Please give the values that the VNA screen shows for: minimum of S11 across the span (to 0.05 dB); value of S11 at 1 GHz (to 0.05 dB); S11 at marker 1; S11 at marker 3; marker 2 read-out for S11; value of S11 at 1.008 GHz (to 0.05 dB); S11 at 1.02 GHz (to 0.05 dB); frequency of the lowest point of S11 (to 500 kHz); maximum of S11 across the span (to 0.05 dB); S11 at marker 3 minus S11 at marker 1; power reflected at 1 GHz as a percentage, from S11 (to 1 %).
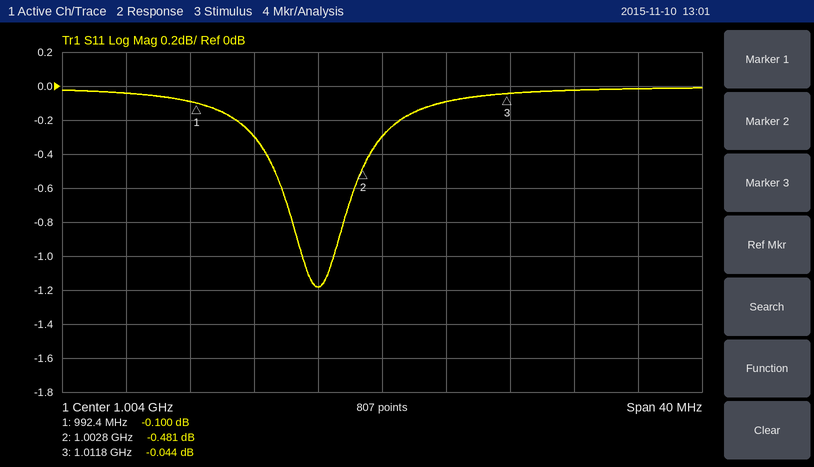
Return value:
-1.20 dB
-1.20 dB
-0.100 dB
-0.044 dB
-0.481 dB
-0.10 dB
0.00 dB
1.0000 GHz
0.00 dB
0.056 dB
76 %
